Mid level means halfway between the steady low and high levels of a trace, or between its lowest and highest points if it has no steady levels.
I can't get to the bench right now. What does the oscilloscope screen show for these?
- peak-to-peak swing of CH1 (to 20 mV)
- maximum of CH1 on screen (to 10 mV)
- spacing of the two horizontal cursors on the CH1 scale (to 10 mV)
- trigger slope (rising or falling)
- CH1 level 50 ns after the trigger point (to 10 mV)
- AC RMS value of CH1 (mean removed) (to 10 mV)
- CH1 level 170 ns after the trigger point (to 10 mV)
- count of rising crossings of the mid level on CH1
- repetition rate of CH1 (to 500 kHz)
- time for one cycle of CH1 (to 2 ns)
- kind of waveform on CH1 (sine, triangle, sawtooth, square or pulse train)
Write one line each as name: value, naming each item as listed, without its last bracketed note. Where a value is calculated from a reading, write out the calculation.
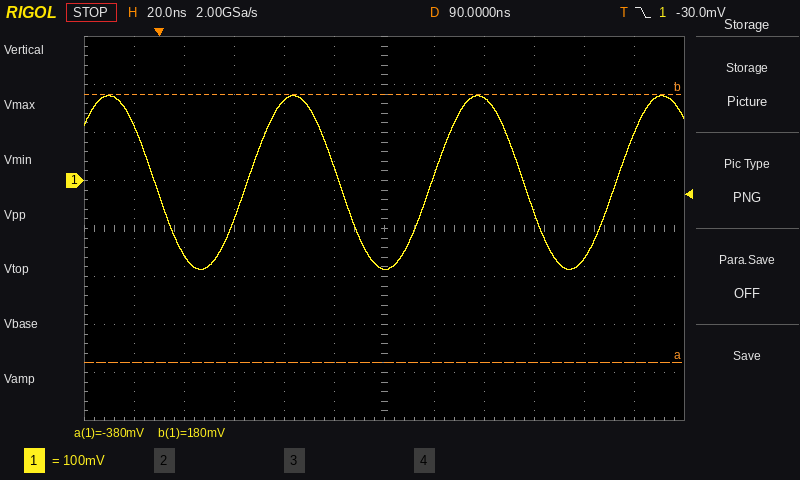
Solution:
peak-to-peak swing of CH1: 360 mV
maximum of CH1 on screen: 180 mV
spacing of the two horizontal cursors on the CH1 scale: 560 mV
trigger slope: falling
CH1 level 50 ns after the trigger point: 170 mV
AC RMS value of CH1 (mean removed): 360 mV / (2√2) ≈ 127 mV, so 130 mV to the nearest 10 mV
CH1 level 170 ns after the trigger point: -160 mV
count of rising crossings of the mid level on CH1: 3
repetition rate of CH1: 1 / 74 ns ≈ 13.5 MHz
time for one cycle of CH1: 74 ns
kind of waveform on CH1: sine
